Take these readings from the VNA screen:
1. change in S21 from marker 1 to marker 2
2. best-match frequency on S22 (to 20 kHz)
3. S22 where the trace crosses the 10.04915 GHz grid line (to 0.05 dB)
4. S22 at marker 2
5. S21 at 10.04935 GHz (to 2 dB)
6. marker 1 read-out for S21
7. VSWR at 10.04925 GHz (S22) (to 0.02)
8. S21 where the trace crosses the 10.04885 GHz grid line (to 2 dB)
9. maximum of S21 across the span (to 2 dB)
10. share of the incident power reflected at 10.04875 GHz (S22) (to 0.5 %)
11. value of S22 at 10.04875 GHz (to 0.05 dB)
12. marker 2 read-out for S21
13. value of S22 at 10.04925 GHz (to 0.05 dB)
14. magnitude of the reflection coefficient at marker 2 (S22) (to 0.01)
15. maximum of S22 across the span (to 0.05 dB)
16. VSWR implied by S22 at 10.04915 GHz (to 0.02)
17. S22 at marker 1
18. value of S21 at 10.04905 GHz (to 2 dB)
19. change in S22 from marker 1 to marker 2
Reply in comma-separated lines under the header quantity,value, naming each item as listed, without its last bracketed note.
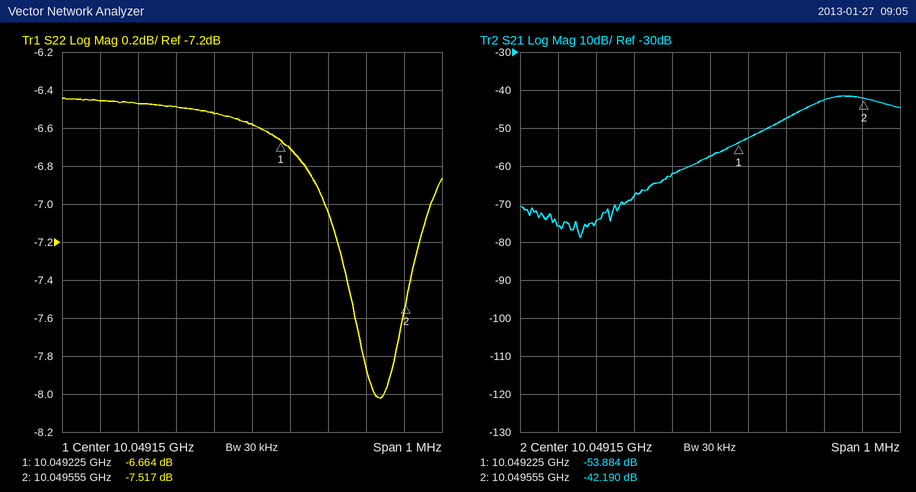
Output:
quantity,value
change in S21 from marker 1 to marker 2,11.694 dB
best-match frequency on S22,10.04948 GHz
S22 where the trace crosses the 10.04915 GHz grid line,-6.60 dB
S22 at marker 2,-7.517 dB
S21 at 10.04935 GHz,-48 dB
marker 1 read-out for S21,-53.884 dB
VSWR at 10.04925 GHz (S22),2.72
S21 where the trace crosses the 10.04885 GHz grid line,-74 dB
maximum of S21 across the span,-42 dB
share of the incident power reflected at 10.04875 GHz (S22),22.5 %
value of S22 at 10.04875 GHz,-6.45 dB
marker 2 read-out for S21,-42.190 dB
value of S22 at 10.04925 GHz,-6.70 dB
magnitude of the reflection coefficient at marker 2 (S22),0.42
maximum of S22 across the span,-6.45 dB
VSWR implied by S22 at 10.04915 GHz,2.76
S22 at marker 1,-6.664 dB
value of S21 at 10.04905 GHz,-62 dB
change in S22 from marker 1 to marker 2,-0.853 dB
